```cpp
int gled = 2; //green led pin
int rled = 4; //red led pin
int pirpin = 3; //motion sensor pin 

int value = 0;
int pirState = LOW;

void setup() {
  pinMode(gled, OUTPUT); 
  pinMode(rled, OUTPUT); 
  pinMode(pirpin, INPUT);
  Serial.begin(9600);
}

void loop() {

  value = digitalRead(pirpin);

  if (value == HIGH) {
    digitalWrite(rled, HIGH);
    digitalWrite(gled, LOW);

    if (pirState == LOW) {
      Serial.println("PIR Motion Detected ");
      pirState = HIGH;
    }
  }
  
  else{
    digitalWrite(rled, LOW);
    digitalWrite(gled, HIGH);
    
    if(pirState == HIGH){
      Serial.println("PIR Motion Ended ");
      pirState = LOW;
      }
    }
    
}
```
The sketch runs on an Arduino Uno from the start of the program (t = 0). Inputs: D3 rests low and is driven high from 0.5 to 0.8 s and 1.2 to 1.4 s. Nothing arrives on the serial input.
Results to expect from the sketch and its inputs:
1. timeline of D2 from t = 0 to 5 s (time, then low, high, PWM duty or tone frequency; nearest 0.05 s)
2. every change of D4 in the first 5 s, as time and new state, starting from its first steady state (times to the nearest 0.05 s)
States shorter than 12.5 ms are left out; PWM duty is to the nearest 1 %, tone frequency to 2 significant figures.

0 s high; 0.5 s low; 0.8 s high; 1.2 s low; 1.4 s high
0 s low; 0.5 s high; 0.8 s low; 1.2 s high; 1.4 s low
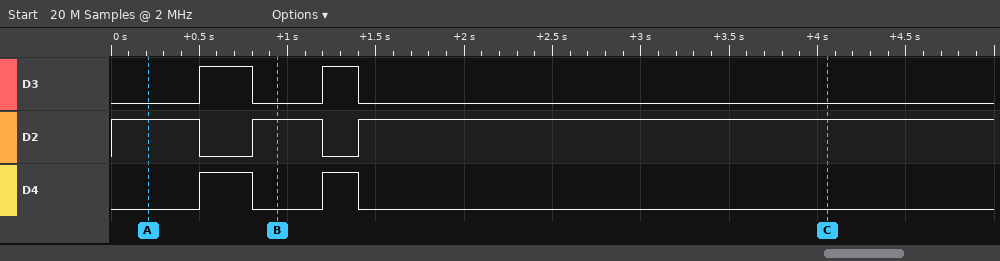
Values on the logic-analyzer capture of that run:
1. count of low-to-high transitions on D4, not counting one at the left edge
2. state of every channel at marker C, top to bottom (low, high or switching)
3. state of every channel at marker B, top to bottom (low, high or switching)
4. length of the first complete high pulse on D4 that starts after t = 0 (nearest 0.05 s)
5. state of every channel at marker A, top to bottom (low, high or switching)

2
D3 low, D2 high, D4 low
D3 low, D2 high, D4 low
0.30 s
D3 low, D2 high, D4 low
